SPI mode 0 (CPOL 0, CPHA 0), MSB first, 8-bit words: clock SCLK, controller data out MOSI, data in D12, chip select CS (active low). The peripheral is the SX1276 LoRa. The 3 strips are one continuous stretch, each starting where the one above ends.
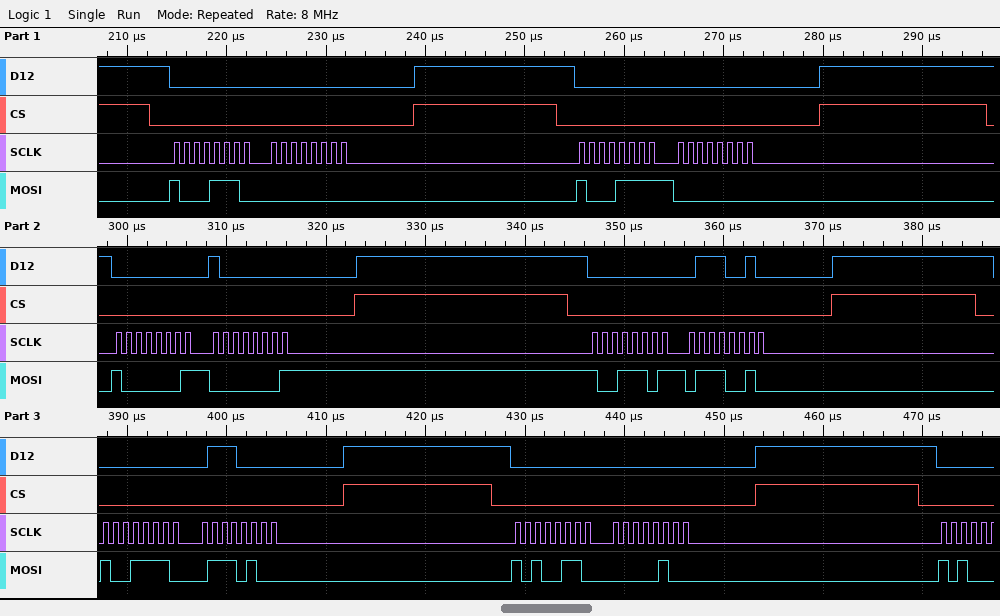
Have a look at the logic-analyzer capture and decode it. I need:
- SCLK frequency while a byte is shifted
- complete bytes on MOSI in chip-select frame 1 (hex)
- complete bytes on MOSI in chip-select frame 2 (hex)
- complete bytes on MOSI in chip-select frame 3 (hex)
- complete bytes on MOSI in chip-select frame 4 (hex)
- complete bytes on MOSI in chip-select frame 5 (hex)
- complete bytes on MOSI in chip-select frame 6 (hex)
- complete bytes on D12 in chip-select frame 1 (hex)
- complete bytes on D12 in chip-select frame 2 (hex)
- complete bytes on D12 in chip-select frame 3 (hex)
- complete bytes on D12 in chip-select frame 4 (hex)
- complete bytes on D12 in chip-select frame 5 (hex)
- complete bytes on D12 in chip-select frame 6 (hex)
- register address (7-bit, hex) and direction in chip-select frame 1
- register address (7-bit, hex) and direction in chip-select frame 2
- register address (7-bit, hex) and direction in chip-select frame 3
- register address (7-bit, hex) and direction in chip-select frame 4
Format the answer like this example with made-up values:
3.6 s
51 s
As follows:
1 MHz
8E 00
8F 00
81 01
9D 72
9E 74
A6 04
00 00
00 00
00 80
00 72
00 70
00 00
0x0E write
0x0F write
0x01 write
0x1D write
